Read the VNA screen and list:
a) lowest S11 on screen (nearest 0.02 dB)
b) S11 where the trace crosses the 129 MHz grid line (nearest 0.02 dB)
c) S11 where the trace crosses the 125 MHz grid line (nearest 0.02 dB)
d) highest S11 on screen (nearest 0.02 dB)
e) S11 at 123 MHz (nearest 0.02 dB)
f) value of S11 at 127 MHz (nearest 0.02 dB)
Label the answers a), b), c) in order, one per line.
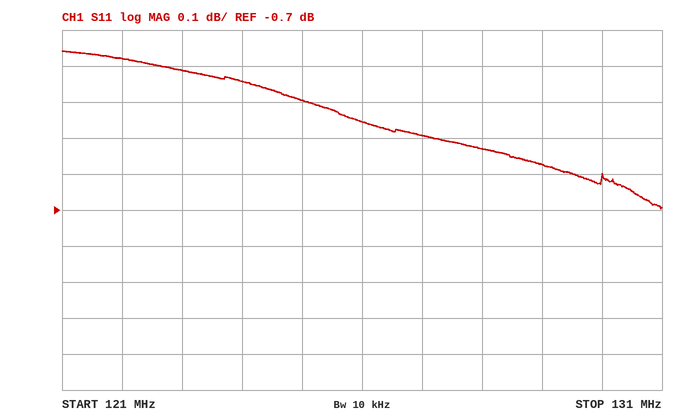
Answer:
a) -0.70 dB
b) -0.58 dB
c) -0.40 dB
d) -0.26 dB
e) -0.32 dB
f) -0.50 dB
